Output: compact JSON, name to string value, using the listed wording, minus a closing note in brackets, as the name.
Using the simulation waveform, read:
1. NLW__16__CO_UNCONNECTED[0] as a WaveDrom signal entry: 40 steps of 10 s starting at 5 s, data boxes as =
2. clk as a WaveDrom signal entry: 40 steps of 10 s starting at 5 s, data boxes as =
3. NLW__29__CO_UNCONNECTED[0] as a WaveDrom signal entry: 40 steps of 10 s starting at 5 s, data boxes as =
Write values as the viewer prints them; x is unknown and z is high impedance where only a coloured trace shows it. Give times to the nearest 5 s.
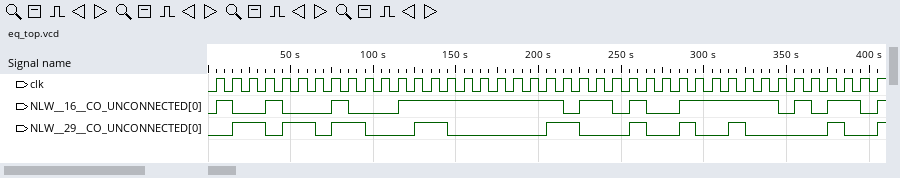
{"NLW__16__CO_UNCONNECTED[0] as a WaveDrom signal entry: 40 steps of 10 s starting at 5 s, data boxes as =": "{name: 'NLW__16__CO_UNCONNECTED[0]', wave: '10.10..10..1.........01.010.1.....0101.0'}", "clk as a WaveDrom signal entry: 40 steps of 10 s starting at 5 s, data boxes as =": "{name: 'clk', wave: 'p.......................................'}", "NLW__29__CO_UNCONNECTED[0] as a WaveDrom signal entry: 40 steps of 10 s starting at 5 s, data boxes as =": "{name: 'NLW__29__CO_UNCONNECTED[0]', wave: '01.01.01.0..1.0.....1.0..10.10.10....10.'}"}
